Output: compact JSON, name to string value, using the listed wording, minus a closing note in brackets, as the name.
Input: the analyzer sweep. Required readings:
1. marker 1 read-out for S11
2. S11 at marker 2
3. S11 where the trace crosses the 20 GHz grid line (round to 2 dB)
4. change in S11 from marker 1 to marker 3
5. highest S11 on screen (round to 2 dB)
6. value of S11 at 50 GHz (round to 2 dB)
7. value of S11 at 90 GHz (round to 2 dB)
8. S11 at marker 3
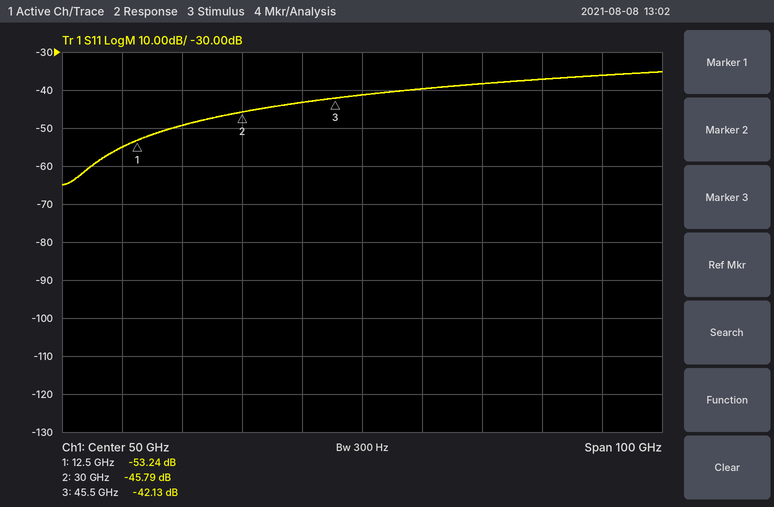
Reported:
{"marker 1 read-out for S11": "-53.24 dB", "S11 at marker 2": "-45.79 dB", "S11 where the trace crosses the 20 GHz grid line": "-50 dB", "change in S11 from marker 1 to marker 3": "11.11 dB", "highest S11 on screen": "-36 dB", "value of S11 at 50 GHz": "-42 dB", "value of S11 at 90 GHz": "-36 dB", "S11 at marker 3": "-42.13 dB"}
